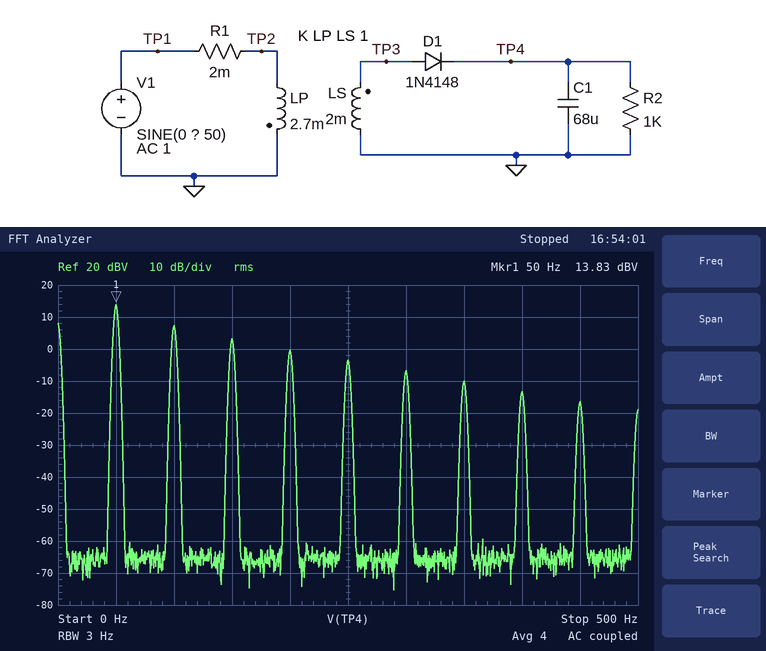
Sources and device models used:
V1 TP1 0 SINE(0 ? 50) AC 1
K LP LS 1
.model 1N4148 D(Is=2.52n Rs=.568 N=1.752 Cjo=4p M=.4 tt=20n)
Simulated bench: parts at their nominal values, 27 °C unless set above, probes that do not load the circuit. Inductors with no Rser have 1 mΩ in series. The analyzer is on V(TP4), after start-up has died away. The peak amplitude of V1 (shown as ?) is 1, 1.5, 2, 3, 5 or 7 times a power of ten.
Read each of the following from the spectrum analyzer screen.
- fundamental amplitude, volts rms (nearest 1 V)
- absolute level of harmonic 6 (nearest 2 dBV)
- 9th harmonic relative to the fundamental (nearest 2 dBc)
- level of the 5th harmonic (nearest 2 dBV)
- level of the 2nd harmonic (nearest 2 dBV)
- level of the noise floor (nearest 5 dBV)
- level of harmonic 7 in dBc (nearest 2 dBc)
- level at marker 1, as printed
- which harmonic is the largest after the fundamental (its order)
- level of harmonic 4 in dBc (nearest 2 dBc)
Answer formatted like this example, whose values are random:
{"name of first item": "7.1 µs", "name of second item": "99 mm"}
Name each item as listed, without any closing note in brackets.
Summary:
{"fundamental amplitude, volts rms": "5 V", "absolute level of harmonic 6": "-6 dBV", "9th harmonic relative to the fundamental": "-30 dBc", "level of the 5th harmonic": "-4 dBV", "level of the 2nd harmonic": "8 dBV", "level of the noise floor": "-65 dBV", "level of harmonic 7 in dBc": "-24 dBc", "level at marker 1, as printed": "13.83 dBV", "which harmonic is the largest after the fundamental": "2", "level of harmonic 4 in dBc": "-14 dBc"}
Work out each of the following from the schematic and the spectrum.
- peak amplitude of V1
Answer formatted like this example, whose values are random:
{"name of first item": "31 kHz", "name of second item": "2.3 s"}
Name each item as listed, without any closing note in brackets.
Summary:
{"peak amplitude of V1": "100 V"}
